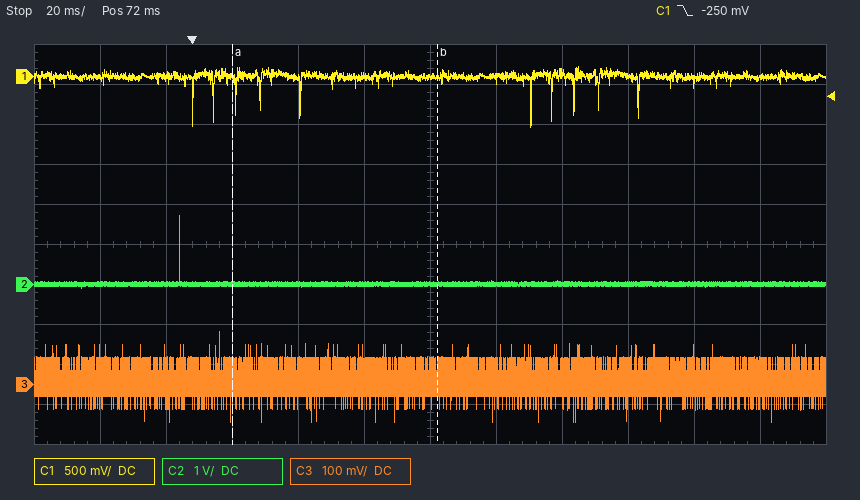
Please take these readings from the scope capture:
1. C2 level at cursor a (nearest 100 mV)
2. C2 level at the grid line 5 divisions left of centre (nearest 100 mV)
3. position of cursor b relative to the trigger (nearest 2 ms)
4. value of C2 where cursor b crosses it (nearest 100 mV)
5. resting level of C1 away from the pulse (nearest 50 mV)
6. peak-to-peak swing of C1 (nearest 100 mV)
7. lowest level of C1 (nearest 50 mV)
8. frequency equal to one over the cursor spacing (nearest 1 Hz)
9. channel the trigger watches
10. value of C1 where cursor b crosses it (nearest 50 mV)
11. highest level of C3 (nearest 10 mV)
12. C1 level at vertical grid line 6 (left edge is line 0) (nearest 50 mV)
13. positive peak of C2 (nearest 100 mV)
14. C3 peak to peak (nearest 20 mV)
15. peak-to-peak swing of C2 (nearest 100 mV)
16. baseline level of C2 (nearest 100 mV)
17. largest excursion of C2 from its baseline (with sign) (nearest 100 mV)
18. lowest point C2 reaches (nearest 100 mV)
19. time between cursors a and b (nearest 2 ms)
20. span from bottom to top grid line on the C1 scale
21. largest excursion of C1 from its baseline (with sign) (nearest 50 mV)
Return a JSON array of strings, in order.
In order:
["0.0 V", "0.0 V", "+74 ms", "0.0 V", "0 mV", "800 mV", "-650 mV", "16 Hz", "C1", "0 mV", "130 mV", "0 mV", "1.7 V", "220 mV", "1.8 V", "0.0 V", "+1.7 V", "-100 mV", "62 ms", "5 V", "-650 mV"]
